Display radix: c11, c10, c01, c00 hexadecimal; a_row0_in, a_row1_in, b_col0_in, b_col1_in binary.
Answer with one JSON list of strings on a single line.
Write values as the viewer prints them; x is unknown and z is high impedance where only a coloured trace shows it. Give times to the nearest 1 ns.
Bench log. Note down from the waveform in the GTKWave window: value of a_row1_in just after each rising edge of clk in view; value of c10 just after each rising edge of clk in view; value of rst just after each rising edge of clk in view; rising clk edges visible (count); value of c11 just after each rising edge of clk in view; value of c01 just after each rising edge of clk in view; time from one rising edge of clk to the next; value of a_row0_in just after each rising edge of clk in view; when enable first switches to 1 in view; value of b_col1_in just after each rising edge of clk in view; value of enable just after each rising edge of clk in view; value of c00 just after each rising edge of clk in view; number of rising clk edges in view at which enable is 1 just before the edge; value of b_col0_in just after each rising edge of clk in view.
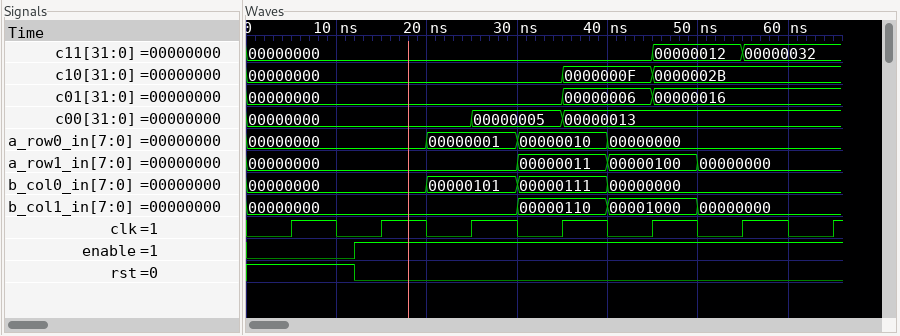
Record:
["00000000, 00000000, 00000000, 00000011, 00000100, 00000000, 00000000", "00000000, 00000000, 00000000, 0000000F, 0000002B, 0000002B, 0000002B", "1 0 0 0 0 0 0", "7", "00000000, 00000000, 00000000, 00000000, 00000012, 00000032, 00000032", "00000000, 00000000, 00000000, 00000006, 00000016, 00000016, 00000016", "10 ns", "00000000, 00000000, 00000001, 00000010, 00000000, 00000000, 00000000", "12 ns", "00000000, 00000000, 00000000, 00000110, 00001000, 00000000, 00000000", "0 1 1 1 1 1 1", "00000000, 00000000, 00000005, 00000013, 00000013, 00000013, 00000013", "6", "00000000, 00000000, 00000101, 00000111, 00000000, 00000000, 00000000"]
